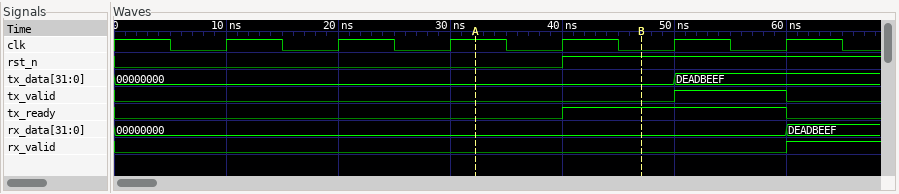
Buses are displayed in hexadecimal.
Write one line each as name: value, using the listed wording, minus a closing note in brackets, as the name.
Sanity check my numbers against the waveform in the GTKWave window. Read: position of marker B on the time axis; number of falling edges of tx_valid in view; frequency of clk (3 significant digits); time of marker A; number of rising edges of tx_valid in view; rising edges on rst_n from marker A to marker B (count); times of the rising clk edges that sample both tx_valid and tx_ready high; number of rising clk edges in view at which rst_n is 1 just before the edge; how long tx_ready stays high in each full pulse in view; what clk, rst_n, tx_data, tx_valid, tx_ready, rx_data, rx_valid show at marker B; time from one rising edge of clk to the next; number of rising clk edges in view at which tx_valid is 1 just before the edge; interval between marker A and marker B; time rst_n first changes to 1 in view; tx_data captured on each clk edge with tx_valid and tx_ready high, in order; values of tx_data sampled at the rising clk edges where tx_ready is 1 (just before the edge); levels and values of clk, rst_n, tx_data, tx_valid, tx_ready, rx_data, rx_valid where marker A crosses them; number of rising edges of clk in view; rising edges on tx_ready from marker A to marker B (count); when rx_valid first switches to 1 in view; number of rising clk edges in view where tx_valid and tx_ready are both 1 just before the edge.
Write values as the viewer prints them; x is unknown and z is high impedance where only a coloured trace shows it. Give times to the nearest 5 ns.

position of marker B on the time axis: 45 ns
number of falling edges of tx_valid in view: 1
frequency of clk: 100 MHz
time of marker A: 30 ns
number of rising edges of tx_valid in view: 1
rising edges on rst_n from marker A to marker B: 1
times of the rising clk edges that sample both tx_valid and tx_ready high: 60 ns
number of rising clk edges in view at which rst_n is 1 just before the edge: 2
how long tx_ready stays high in each full pulse in view: 20 ns
what clk, rst_n, tx_data, tx_valid, tx_ready, rx_data, rx_valid show at marker B: clk=0, rst_n=1, tx_data=00000000, tx_valid=0, tx_ready=1, rx_data=00000000, rx_valid=0
time from one rising edge of clk to the next: 10 ns
number of rising clk edges in view at which tx_valid is 1 just before the edge: 1
interval between marker A and marker B: 15 ns
time rst_n first changes to 1 in view: 40 ns
tx_data captured on each clk edge with tx_valid and tx_ready high, in order: DEADBEEF
values of tx_data sampled at the rising clk edges where tx_ready is 1: 00000000, DEADBEEF
levels and values of clk, rst_n, tx_data, tx_valid, tx_ready, rx_data, rx_valid where marker A crosses them: clk=1, rst_n=0, tx_data=00000000, tx_valid=0, tx_ready=0, rx_data=00000000, rx_valid=0
number of rising edges of clk in view: 6
rising edges on tx_ready from marker A to marker B: 1
when rx_valid first switches to 1 in view: 60 ns
number of rising clk edges in view where tx_valid and tx_ready are both 1 just before the edge: 1
